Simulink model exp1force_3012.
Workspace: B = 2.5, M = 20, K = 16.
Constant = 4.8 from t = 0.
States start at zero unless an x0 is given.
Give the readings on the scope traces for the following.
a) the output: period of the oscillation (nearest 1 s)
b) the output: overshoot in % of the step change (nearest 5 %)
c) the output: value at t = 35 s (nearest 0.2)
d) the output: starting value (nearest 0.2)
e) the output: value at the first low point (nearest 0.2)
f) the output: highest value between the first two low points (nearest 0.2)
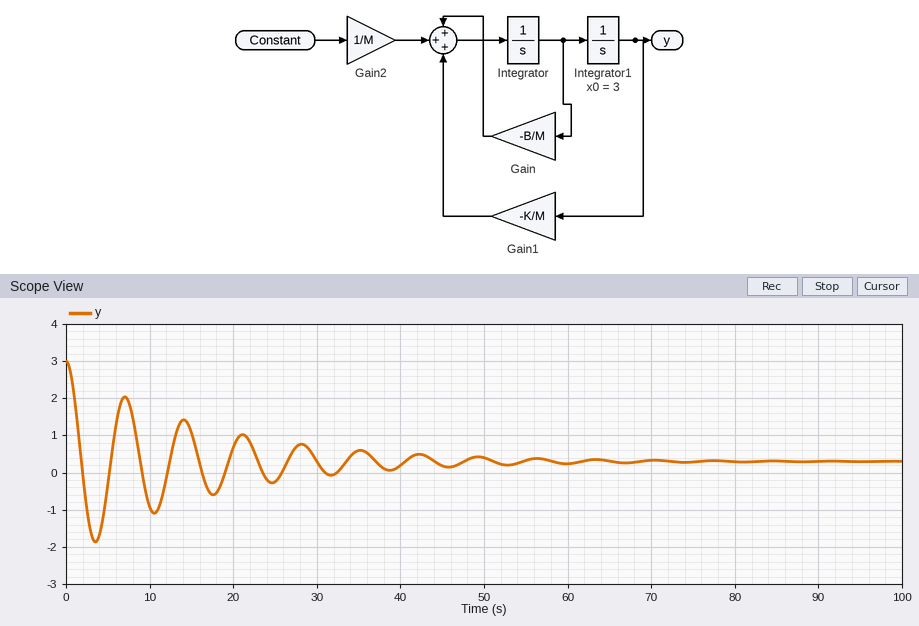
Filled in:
7 s
80 %
0.6
3.0
-1.8
2.0
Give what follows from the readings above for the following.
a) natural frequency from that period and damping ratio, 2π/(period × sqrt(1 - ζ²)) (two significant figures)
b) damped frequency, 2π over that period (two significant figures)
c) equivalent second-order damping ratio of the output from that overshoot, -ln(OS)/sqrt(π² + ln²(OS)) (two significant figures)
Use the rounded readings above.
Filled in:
0.90 rad/s
0.90 rad/s
0.071
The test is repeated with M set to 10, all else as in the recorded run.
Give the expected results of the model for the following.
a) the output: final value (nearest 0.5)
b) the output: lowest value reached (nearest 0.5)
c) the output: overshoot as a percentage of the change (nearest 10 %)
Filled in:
0.5
-1.5
70 %
